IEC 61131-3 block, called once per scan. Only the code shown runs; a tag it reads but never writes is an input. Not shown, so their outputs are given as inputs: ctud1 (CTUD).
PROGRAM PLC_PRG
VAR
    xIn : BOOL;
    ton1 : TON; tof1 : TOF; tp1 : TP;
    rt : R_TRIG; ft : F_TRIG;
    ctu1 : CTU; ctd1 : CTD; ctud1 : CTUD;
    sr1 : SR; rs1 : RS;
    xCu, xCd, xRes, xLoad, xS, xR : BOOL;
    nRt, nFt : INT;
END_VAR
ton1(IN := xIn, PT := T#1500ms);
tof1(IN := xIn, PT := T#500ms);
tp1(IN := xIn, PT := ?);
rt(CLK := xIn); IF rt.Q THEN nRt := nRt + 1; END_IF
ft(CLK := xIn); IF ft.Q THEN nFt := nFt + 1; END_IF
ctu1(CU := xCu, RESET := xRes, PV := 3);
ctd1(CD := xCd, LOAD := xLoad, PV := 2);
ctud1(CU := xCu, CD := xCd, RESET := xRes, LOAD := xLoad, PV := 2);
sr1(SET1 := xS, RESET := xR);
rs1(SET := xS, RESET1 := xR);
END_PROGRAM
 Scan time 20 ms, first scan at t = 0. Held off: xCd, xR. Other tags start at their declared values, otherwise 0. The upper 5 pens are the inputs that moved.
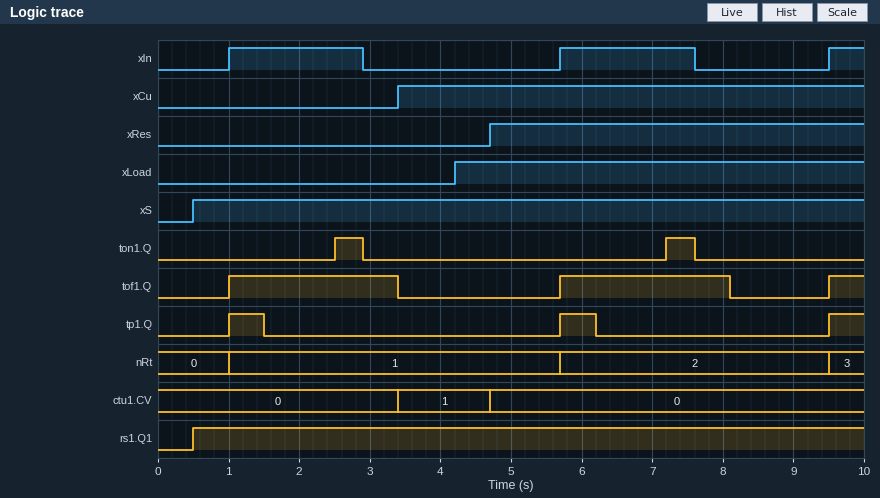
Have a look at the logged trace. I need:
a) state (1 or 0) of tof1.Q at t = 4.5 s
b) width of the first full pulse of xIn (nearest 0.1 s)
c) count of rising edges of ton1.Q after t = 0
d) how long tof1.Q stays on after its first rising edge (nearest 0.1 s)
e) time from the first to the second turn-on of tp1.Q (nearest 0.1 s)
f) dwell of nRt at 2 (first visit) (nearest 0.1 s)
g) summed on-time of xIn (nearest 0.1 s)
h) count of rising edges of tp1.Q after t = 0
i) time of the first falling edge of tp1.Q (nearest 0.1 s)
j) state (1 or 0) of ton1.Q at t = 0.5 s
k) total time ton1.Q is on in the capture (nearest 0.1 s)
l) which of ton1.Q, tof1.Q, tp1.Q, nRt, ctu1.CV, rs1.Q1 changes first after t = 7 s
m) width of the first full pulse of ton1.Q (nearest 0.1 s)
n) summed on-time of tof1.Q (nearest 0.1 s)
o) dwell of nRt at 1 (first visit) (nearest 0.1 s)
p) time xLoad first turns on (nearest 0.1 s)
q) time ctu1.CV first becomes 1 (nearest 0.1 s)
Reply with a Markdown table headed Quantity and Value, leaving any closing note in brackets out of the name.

| Quantity | Value |
|---|---|
| state (1 or 0) of tof1.Q at t = 4.5 s | 0 |
| width of the first full pulse of xIn | 1.9 s |
| count of rising edges of ton1.Q after t = 0 | 2 |
| how long tof1.Q stays on after its first rising edge | 2.4 s |
| time from the first to the second turn-on of tp1.Q | 4.7 s |
| dwell of nRt at 2 (first visit) | 3.8 s |
| summed on-time of xIn | 4.3 s |
| count of rising edges of tp1.Q after t = 0 | 3 |
| time of the first falling edge of tp1.Q | 1.5 s |
| state (1 or 0) of ton1.Q at t = 0.5 s | 0 |
| total time ton1.Q is on in the capture | 0.8 s |
| which of ton1.Q, tof1.Q, tp1.Q, nRt, ctu1.CV, rs1.Q1 changes first after t = 7 s | ton1.Q |
| width of the first full pulse of ton1.Q | 0.4 s |
| summed on-time of tof1.Q | 5.3 s |
| dwell of nRt at 1 (first visit) | 4.7 s |
| time xLoad first turns on | 4.2 s |
| time ctu1.CV first becomes 1 | 3.4 s |
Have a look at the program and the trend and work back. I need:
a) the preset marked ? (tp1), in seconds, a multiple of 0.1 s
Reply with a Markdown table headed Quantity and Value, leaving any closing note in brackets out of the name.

| Quantity | Value |
|---|---|
| the preset marked ? (tp1), in seconds, a multiple of 0.1 s | 0.5 s |
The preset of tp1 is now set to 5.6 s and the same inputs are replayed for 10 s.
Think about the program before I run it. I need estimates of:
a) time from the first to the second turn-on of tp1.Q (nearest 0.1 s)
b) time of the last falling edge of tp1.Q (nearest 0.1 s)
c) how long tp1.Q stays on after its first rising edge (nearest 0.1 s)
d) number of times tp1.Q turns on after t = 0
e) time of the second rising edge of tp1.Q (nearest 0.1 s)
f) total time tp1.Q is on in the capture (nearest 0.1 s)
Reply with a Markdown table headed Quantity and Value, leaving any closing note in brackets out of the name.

| Quantity | Value |
|---|---|
| time from the first to the second turn-on of tp1.Q | 8.5 s |
| time of the last falling edge of tp1.Q | 6.6 s |
| how long tp1.Q stays on after its first rising edge | 5.6 s |
| number of times tp1.Q turns on after t = 0 | 2 |
| time of the second rising edge of tp1.Q | 9.5 s |
| total time tp1.Q is on in the capture | 6.1 s |
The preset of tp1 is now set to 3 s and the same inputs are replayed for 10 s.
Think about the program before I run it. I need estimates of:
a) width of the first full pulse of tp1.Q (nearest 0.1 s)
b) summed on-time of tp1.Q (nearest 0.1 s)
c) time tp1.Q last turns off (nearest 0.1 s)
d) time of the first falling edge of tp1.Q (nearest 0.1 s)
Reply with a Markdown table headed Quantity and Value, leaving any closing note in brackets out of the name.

| Quantity | Value |
|---|---|
| width of the first full pulse of tp1.Q | 3.0 s |
| summed on-time of tp1.Q | 6.5 s |
| time tp1.Q last turns off | 8.7 s |
| time of the first falling edge of tp1.Q | 4.0 s |
